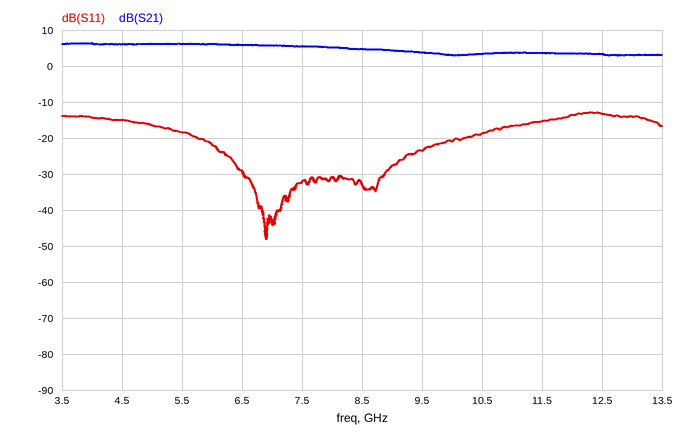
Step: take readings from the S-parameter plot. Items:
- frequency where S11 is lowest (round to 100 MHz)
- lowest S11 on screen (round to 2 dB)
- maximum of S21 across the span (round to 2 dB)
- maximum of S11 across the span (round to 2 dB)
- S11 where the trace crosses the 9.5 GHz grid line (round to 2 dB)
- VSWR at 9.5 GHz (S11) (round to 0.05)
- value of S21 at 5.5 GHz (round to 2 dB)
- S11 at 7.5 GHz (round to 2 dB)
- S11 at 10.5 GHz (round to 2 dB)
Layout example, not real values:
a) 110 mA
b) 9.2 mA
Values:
a) 6.9 GHz
b) -48 dB
c) 6 dB
d) -12 dB
e) -24 dB
f) 1.15
g) 6 dB
h) -32 dB
i) -18 dB
